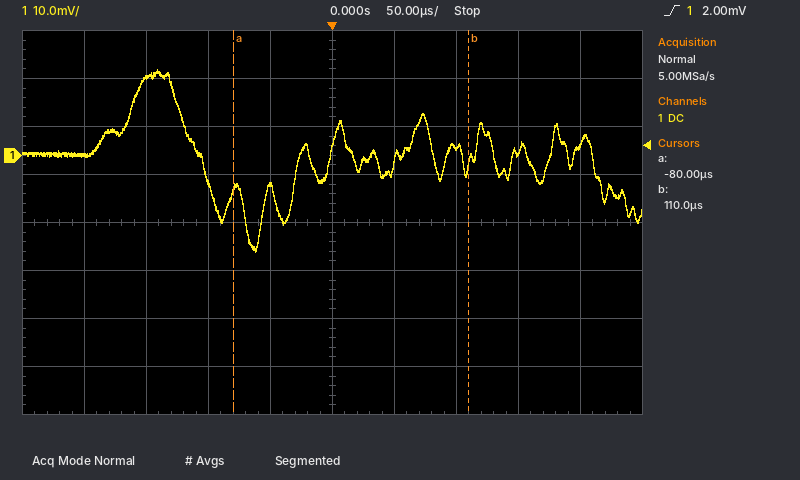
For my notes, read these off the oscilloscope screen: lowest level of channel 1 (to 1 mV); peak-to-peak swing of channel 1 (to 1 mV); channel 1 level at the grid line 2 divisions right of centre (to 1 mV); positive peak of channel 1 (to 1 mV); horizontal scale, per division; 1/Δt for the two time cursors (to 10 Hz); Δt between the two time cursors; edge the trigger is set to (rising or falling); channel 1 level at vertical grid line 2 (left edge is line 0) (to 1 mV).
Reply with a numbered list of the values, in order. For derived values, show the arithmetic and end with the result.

1. -20 mV
2. 18 mV − (-20 mV) = 38 mV
3. 2 mV
4. 18 mV
5. 50 µs
6. 1 / 190 µs ≈ 5.26 kHz
7. 110 µs − (-80 µs) = 190 µs
8. rising
9. 16 mV
